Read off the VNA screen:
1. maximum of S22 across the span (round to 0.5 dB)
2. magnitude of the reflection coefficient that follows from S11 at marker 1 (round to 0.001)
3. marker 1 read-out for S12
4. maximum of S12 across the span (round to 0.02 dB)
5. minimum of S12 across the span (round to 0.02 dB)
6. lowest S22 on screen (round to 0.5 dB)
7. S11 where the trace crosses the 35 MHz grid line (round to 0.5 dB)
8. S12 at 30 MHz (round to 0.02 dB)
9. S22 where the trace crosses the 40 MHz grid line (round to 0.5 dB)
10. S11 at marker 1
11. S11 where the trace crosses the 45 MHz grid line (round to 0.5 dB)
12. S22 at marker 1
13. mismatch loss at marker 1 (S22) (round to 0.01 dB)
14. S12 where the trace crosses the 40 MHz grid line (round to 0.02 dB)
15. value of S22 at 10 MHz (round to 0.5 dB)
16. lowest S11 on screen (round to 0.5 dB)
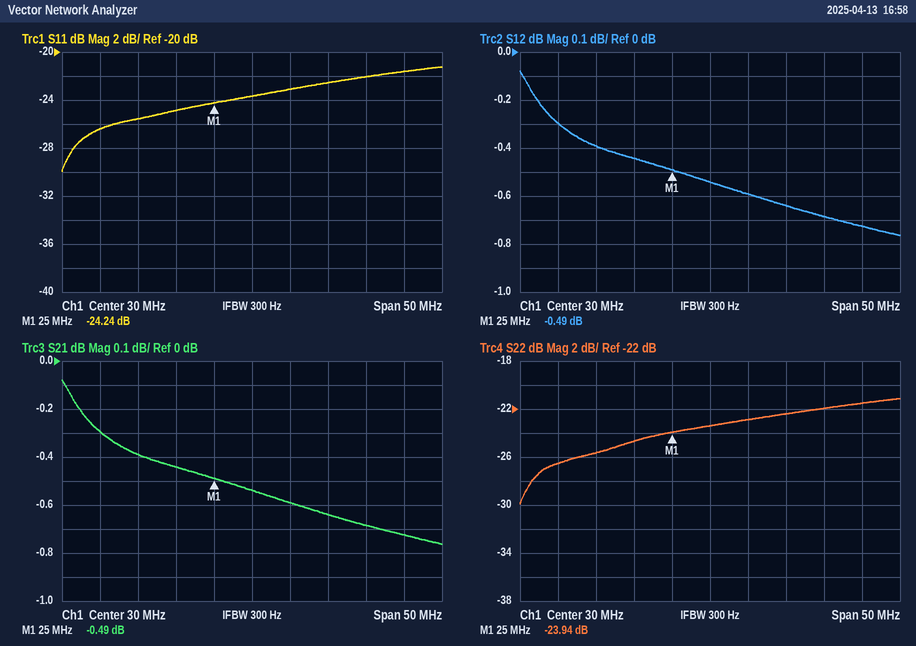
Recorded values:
-21.0 dB
0.061
-0.49 dB
-0.08 dB
-0.76 dB
-30.0 dB
-23.0 dB
-0.54 dB
-22.5 dB
-24.24 dB
-22.0 dB
-23.94 dB
0.02 dB
-0.64 dB
-26.5 dB
-30.0 dB
